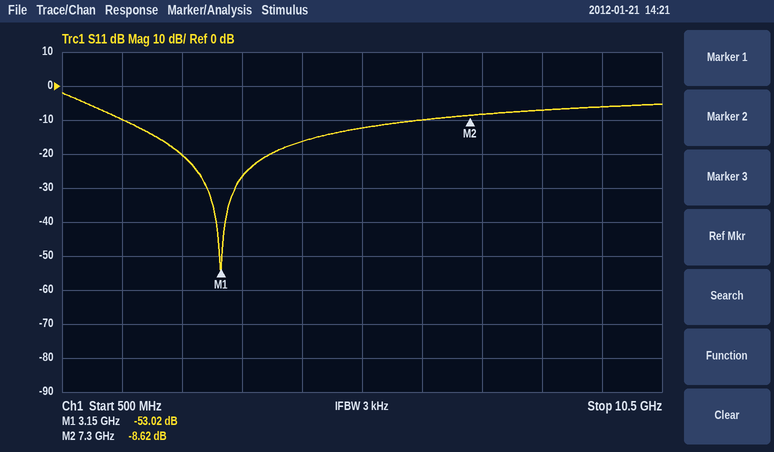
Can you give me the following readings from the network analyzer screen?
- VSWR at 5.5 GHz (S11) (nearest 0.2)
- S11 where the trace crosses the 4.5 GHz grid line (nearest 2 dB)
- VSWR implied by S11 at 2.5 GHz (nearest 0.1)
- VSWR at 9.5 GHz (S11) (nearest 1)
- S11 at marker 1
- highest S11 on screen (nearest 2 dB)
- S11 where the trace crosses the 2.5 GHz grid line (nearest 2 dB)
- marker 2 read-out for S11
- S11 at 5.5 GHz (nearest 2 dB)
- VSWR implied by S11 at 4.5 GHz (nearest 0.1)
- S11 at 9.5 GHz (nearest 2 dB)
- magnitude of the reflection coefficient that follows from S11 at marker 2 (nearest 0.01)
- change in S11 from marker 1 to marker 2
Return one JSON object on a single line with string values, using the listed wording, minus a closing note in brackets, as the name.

{"VSWR at 5.5 GHz (S11)": "1.6", "S11 where the trace crosses the 4.5 GHz grid line": "-16 dB", "VSWR implied by S11 at 2.5 GHz": "1.2", "VSWR at 9.5 GHz (S11)": "3", "S11 at marker 1": "-53.02 dB", "highest S11 on screen": "-2 dB", "S11 where the trace crosses the 2.5 GHz grid line": "-20 dB", "marker 2 read-out for S11": "-8.62 dB", "S11 at 5.5 GHz": "-12 dB", "VSWR implied by S11 at 4.5 GHz": "1.4", "S11 at 9.5 GHz": "-6 dB", "magnitude of the reflection coefficient that follows from S11 at marker 2": "0.37", "change in S11 from marker 1 to marker 2": "44.40 dB"}
